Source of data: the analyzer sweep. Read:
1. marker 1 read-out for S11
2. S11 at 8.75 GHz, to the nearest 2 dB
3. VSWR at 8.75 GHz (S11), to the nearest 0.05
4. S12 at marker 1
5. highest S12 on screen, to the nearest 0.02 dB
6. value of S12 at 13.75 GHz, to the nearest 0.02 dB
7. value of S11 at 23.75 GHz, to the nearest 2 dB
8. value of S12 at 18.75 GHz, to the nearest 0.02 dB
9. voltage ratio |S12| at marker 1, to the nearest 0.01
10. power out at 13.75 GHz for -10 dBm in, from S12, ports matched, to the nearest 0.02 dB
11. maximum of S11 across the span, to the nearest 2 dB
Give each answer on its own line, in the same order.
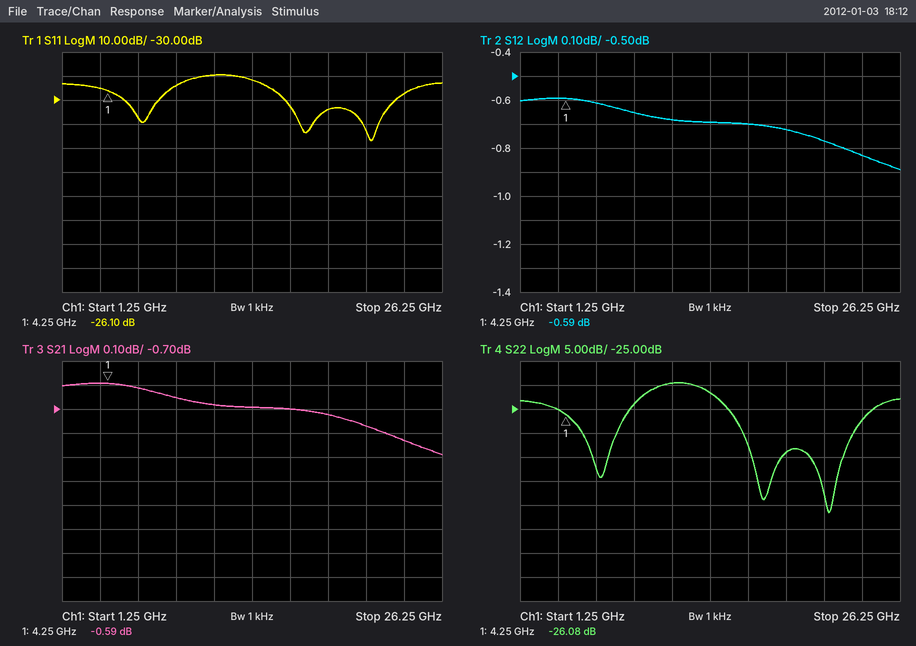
-26.10 dB
-24 dB
1.15
-0.59 dB
-0.60 dB
-0.70 dB
-28 dB
-0.72 dB
0.93
-10.70 dBm
-20 dB
